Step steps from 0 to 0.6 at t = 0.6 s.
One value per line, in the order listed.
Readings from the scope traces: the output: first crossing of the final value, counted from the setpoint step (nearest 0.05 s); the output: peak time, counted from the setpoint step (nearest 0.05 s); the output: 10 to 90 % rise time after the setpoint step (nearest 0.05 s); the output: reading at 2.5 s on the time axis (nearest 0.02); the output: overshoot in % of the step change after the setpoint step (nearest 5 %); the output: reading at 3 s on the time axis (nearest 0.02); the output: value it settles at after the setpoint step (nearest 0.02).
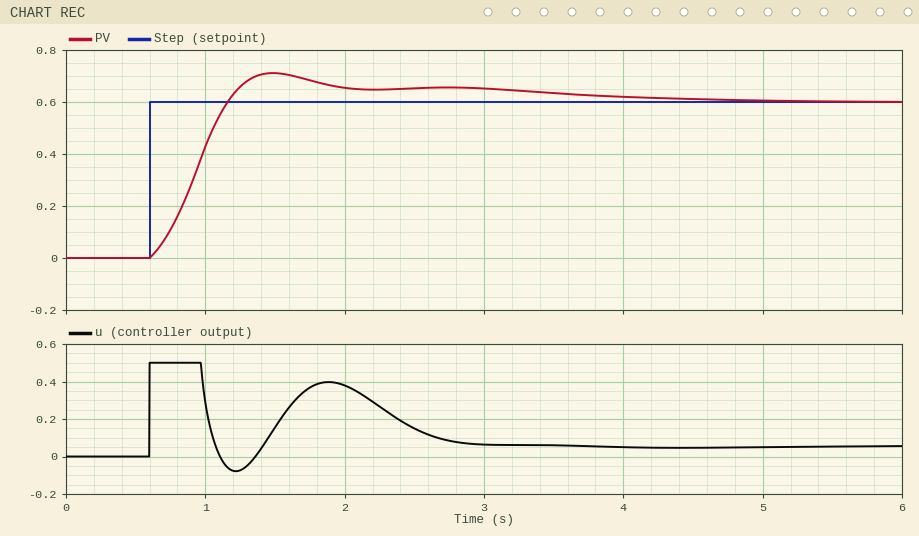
0.55 s
0.90 s
0.40 s
0.66
20 %
0.66
0.60
